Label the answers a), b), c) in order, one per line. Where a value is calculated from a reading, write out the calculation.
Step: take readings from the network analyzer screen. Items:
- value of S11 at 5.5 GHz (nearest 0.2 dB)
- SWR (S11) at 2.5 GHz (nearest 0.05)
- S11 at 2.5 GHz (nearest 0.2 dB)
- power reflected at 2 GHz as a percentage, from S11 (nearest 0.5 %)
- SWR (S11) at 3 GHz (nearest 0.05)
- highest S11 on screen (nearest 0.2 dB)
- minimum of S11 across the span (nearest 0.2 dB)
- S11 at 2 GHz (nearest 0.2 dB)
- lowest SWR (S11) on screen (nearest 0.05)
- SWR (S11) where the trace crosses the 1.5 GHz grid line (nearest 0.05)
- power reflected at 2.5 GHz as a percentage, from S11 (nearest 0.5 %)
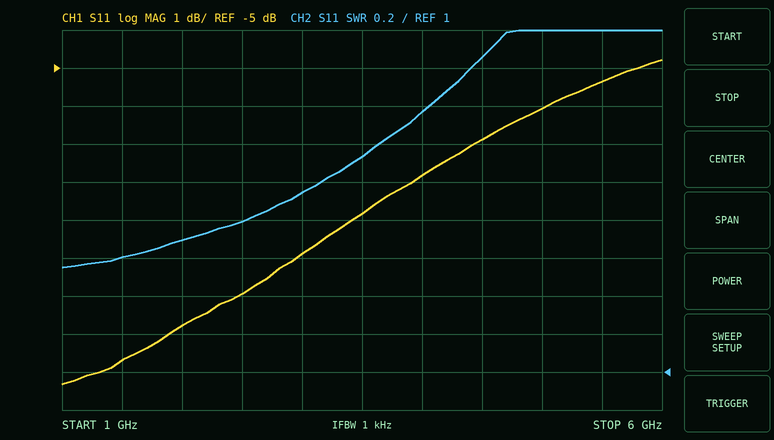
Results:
a) -5.4 dB
b) 1.80
c) -11.0 dB
d) 10^(-11.8/10) ≈ 6.61 %, so 6.5 % to the nearest 0.5 %
e) 1.95
f) -4.8 dB
g) -13.4 dB
h) -11.8 dB
i) 1.55
j) 1.60
k) 10^(-11/10) ≈ 7.94 %, so 8.0 % to the nearest 0.5 %
